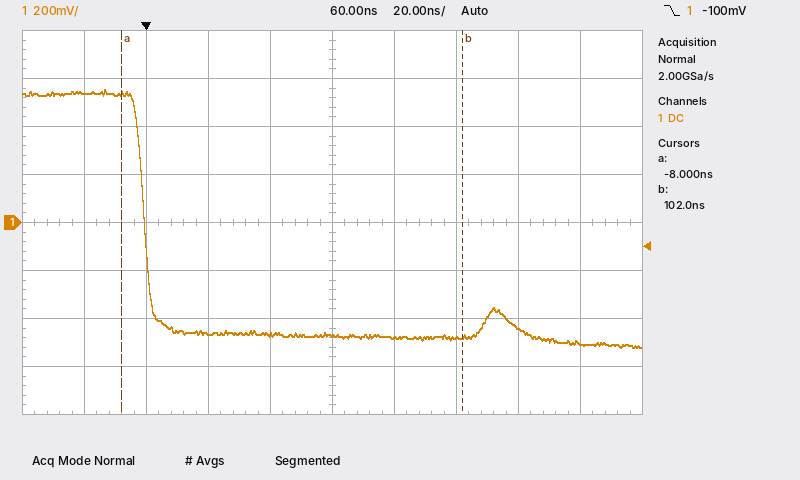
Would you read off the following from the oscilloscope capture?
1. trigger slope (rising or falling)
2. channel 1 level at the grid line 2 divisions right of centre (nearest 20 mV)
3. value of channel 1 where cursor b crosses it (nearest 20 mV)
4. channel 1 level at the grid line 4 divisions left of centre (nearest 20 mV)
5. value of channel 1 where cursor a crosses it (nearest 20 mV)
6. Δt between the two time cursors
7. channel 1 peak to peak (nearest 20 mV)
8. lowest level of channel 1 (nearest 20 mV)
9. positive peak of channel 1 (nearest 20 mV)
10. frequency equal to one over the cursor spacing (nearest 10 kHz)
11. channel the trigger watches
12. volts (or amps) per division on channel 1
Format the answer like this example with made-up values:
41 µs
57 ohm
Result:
falling
-480 mV
-480 mV
540 mV
540 mV
110 ns
1.08 V
-520 mV
560 mV
9.09 MHz
channel 1
200 mV
